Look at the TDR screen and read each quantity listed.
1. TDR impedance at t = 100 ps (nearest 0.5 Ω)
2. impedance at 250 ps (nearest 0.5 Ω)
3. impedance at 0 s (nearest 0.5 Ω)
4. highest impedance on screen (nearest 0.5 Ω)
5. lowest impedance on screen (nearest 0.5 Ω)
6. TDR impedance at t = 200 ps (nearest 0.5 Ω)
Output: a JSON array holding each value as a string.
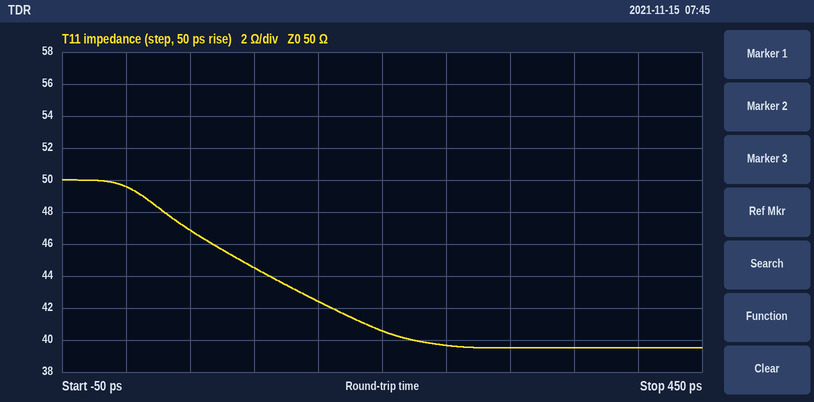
["44.5 Ω", "39.5 Ω", "49.5 Ω", "50.0 Ω", "39.5 Ω", "40.5 Ω"]
